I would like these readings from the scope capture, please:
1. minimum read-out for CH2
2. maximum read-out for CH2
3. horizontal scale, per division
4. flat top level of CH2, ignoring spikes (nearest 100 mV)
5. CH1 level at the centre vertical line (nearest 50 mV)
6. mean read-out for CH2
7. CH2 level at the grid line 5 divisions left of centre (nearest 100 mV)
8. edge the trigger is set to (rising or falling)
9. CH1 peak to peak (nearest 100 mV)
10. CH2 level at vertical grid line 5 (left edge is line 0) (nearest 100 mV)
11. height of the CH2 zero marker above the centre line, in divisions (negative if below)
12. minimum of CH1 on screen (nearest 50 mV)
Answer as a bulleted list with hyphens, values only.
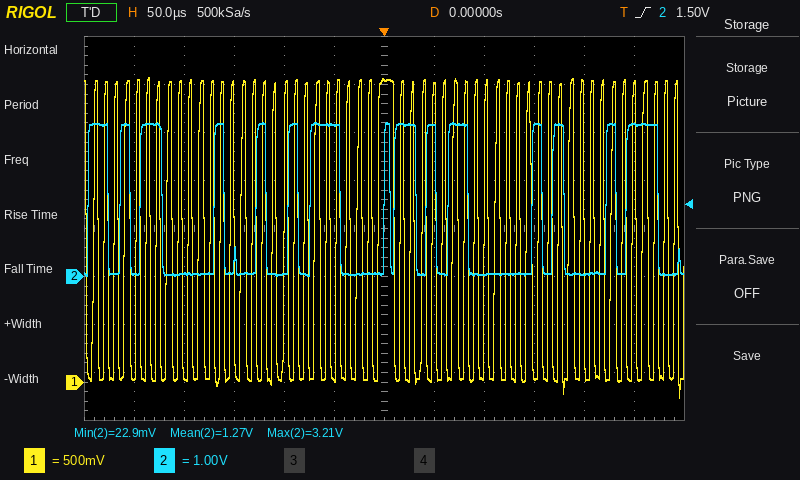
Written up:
- 22.9 mV
- 3.21 V
- 50 µs
- 3.2 V
- 3.15 V
- 1.27 V
- 100 mV
- rising
- 3.30 V
- 3.2 V
- -1.0 div
- -150 mV
